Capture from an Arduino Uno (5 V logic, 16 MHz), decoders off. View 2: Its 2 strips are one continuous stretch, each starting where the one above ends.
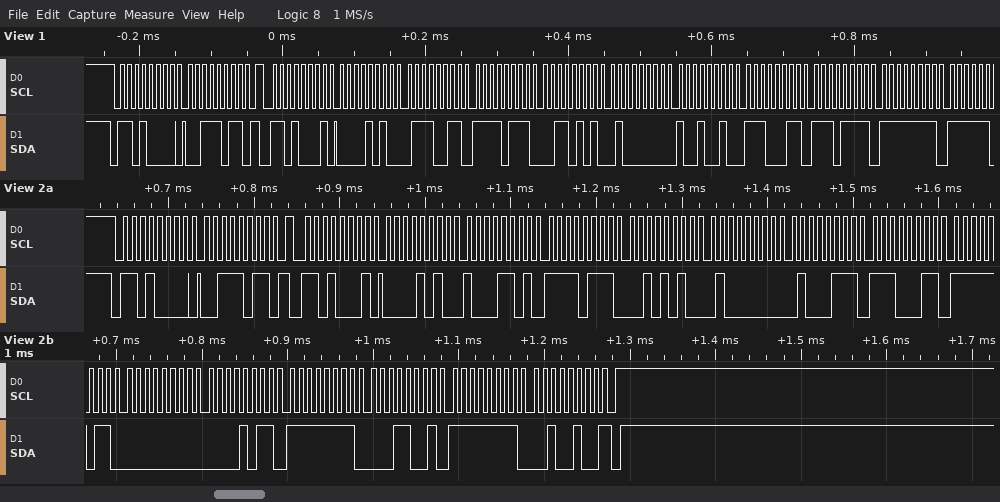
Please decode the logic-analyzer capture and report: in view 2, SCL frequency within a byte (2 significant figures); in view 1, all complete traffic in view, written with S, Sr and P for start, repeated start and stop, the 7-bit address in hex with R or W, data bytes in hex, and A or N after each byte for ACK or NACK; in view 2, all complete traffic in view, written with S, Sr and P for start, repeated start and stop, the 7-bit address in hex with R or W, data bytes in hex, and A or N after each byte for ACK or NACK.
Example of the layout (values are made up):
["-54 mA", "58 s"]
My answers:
["100 kHz", "S 68W A 3B A Sr 68R A 0A A 73 A F7 A 35 A 40 A 92 A E3 A EF A FF A", "S 68W A 3B A Sr 68R A 0A A 8D A F7 A 2A A 40 A 47 A E3 A FB A 00 A 0B A FF A 19 A FF A 24 N P"]
